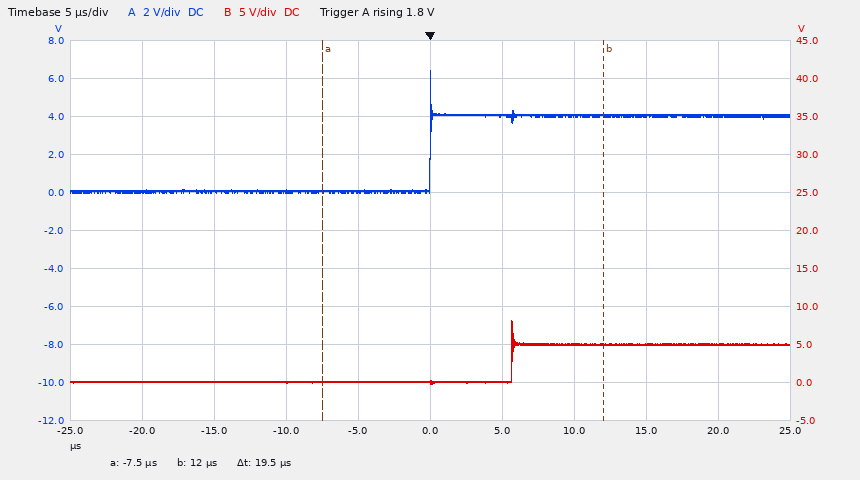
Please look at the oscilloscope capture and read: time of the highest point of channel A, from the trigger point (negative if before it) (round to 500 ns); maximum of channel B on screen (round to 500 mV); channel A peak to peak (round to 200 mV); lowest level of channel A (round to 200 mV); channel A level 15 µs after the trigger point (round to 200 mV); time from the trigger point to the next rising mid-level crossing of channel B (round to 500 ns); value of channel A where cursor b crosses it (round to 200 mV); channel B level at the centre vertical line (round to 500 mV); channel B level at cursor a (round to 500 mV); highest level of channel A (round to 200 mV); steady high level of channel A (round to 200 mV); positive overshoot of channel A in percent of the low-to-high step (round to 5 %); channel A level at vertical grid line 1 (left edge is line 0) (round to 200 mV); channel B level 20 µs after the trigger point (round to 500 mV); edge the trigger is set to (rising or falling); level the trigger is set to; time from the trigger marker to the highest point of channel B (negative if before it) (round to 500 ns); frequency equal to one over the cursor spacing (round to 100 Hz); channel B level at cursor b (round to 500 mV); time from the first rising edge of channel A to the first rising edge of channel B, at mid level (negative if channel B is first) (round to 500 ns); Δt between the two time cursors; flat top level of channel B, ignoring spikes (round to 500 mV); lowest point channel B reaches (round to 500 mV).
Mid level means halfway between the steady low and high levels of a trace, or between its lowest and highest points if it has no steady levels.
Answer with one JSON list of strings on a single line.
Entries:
["0.0 µs", "8.0 V", "6.4 V", "0.0 V", "4.0 V", "5.5 µs", "4.0 V", "0.0 V", "0.0 V", "6.4 V", "4.0 V", "60 %", "0.0 V", "5.0 V", "rising", "1.8 V", "+5.5 µs", "51.3 kHz", "5.0 V", "+5.5 µs", "19.5 µs", "5.0 V", "0.0 V"]
